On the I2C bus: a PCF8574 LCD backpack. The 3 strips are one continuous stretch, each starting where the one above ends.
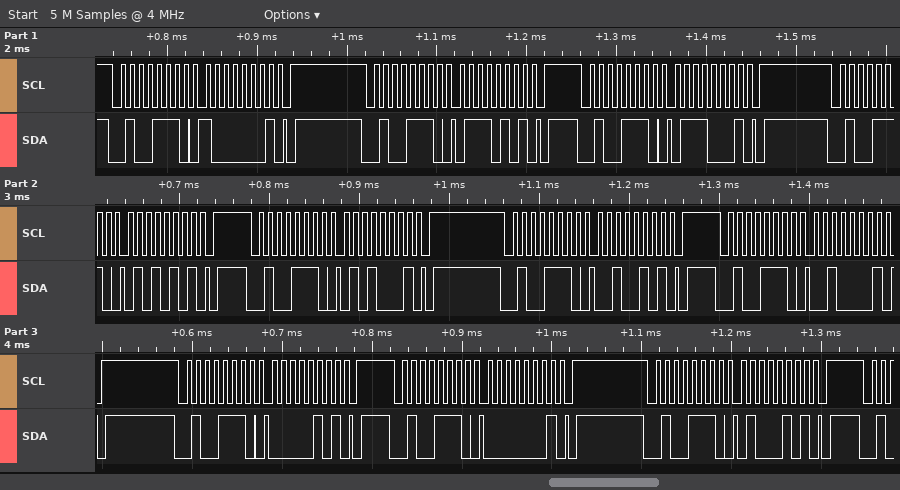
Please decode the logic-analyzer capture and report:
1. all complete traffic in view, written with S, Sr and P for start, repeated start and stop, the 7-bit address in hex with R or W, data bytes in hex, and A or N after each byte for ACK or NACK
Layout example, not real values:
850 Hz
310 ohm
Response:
S 27W A 81 A P S 27W A 75 A P S 27W A 71 A P S 27W A 55 A P S 27W A 51 A P S 27W A 25 A P S 27W A 21 A P S 27W A 05 A P S 27W A 01 A P S 27W A 45 A P
